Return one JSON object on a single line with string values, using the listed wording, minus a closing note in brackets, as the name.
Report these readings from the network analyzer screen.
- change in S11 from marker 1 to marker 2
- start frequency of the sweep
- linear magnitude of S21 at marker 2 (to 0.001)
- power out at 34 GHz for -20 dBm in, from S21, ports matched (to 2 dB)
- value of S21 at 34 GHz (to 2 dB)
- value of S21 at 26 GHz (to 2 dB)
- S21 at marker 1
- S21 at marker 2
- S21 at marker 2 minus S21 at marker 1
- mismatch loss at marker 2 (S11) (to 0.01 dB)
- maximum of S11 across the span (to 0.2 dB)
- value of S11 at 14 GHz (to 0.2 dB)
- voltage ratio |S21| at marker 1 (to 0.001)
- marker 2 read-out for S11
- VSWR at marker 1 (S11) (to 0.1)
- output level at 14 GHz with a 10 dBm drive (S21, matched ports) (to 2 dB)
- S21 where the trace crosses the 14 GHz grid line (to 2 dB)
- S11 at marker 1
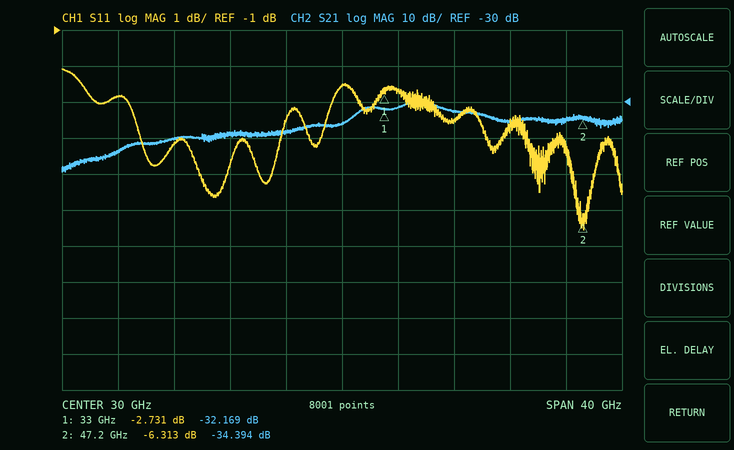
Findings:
{"change in S11 from marker 1 to marker 2": "-3.582 dB", "start frequency of the sweep": "10 GHz", "linear magnitude of S21 at marker 2": "0.019", "power out at 34 GHz for -20 dBm in, from S21, ports matched": "-52 dBm", "value of S21 at 34 GHz": "-32 dB", "value of S21 at 26 GHz": "-38 dB", "S21 at marker 1": "-32.169 dB", "S21 at marker 2": "-34.394 dB", "S21 at marker 2 minus S21 at marker 1": "-2.225 dB", "mismatch loss at marker 2 (S11)": "1.16 dB", "maximum of S11 across the span": "-2.0 dB", "value of S11 at 14 GHz": "-2.8 dB", "voltage ratio |S21| at marker 1": "0.025", "marker 2 read-out for S11": "-6.313 dB", "VSWR at marker 1 (S11)": "6.4", "output level at 14 GHz with a 10 dBm drive (S21, matched ports)": "-34 dBm", "S21 where the trace crosses the 14 GHz grid line": "-44 dB", "S11 at marker 1": "-2.731 dB"}
